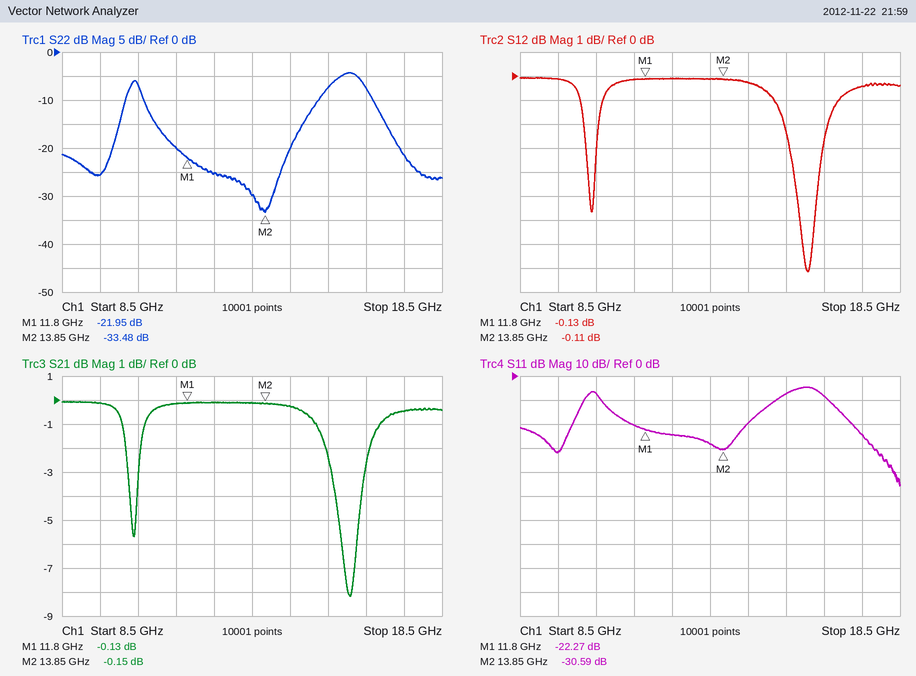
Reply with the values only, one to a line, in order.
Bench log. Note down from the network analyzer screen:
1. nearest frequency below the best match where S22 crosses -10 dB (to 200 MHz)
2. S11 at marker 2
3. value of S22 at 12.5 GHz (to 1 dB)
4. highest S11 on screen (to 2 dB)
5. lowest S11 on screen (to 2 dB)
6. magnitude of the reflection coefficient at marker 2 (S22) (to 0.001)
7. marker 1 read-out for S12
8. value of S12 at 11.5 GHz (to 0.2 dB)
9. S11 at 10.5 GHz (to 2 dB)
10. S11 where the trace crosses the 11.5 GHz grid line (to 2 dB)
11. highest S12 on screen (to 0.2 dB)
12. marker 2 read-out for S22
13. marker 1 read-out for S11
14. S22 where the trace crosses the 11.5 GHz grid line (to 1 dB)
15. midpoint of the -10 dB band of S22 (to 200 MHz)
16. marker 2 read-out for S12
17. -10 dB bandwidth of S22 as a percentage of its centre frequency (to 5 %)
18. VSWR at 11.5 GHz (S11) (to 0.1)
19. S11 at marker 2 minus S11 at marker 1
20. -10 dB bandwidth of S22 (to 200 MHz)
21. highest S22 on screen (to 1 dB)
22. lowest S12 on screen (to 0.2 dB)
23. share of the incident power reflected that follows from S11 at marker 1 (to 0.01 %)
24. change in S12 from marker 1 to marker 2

10.6 GHz
-30.59 dB
-25 dB
-4 dB
-46 dB
0.021
-0.13 dB
-0.2 dB
-8 dB
-20 dB
0.0 dB
-33.48 dB
-22.27 dB
-20 dB
13.0 GHz
-0.11 dB
35 %
1.2
-8.32 dB
4.6 GHz
-4 dB
-8.2 dB
0.59 %
0.02 dB
